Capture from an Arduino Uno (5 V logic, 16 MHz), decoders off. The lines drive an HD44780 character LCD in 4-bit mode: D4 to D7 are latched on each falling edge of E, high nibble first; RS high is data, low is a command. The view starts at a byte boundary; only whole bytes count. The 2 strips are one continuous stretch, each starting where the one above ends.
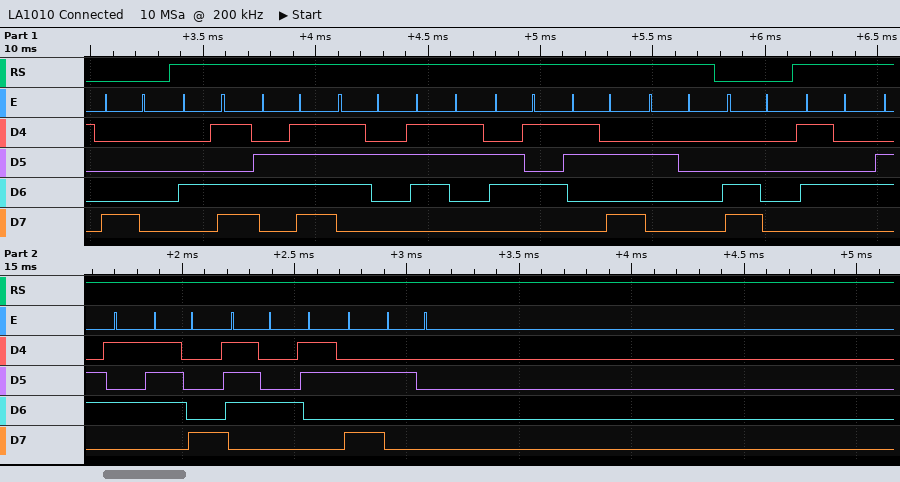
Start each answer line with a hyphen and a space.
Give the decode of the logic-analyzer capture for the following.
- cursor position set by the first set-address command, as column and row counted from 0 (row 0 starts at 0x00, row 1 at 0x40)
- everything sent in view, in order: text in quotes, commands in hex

- column 0, row 0
- 0x80 "Morse: " 0xC0 "Text: "
